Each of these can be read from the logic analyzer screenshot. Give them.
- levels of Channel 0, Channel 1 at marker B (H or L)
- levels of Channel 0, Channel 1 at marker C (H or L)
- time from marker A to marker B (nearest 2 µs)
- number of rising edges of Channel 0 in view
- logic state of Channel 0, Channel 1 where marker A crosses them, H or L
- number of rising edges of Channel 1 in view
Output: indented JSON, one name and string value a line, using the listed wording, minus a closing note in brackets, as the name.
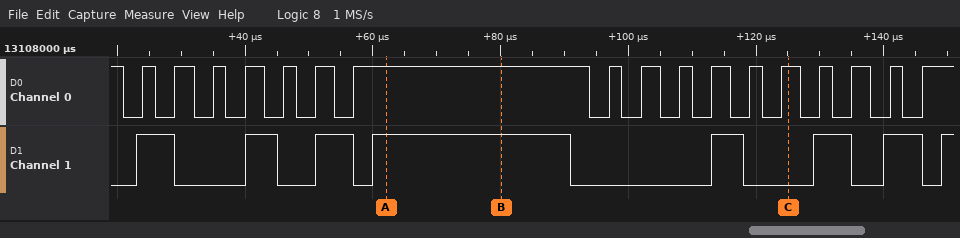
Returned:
{
  "levels of Channel 0, Channel 1 at marker B": "Channel 0=H, Channel 1=H",
  "levels of Channel 0, Channel 1 at marker C": "Channel 0=H, Channel 1=L",
  "time from marker A to marker B": "18 µs",
  "number of rising edges of Channel 0 in view": "17",
  "logic state of Channel 0, Channel 1 where marker A crosses them, H or L": "Channel 0=H, Channel 1=H",
  "number of rising edges of Channel 1 in view": "8"
}
